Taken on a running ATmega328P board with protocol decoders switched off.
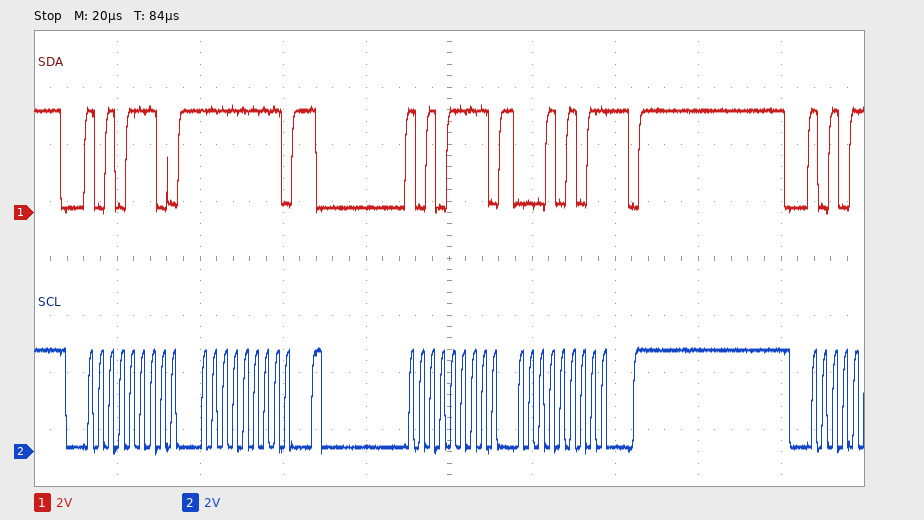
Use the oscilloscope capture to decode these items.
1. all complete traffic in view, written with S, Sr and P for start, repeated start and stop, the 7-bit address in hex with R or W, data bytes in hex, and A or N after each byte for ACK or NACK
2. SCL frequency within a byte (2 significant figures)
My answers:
S 57W A FF A Sr 57R A 15 N P
400 kHz
